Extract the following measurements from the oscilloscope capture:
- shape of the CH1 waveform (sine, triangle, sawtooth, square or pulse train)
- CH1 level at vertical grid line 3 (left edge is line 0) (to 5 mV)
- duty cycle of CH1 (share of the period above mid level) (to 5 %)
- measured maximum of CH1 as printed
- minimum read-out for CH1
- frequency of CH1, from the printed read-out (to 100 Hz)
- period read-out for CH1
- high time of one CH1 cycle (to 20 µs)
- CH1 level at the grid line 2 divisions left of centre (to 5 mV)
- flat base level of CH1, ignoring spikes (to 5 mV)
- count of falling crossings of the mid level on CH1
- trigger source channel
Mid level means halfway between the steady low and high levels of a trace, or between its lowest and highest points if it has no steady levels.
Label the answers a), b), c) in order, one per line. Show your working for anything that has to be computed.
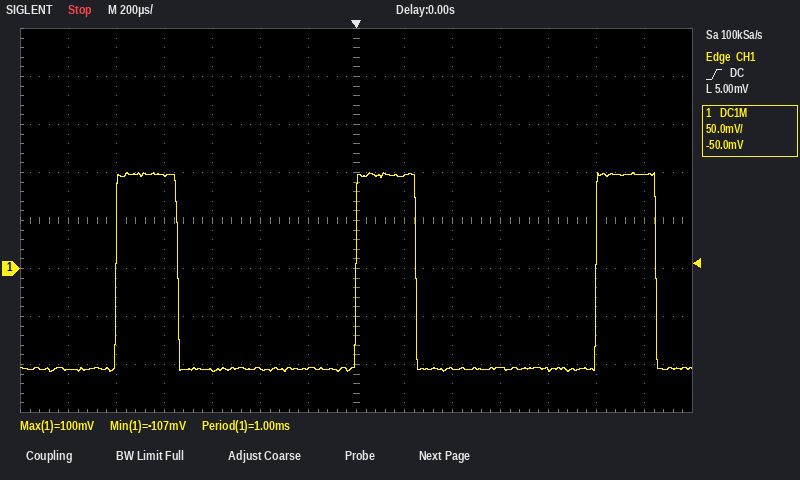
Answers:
a) pulse train
b) 95 mV
c) 25 %
d) 100 mV
e) -107 mV
f) 1 / 1.00 ms ≈ 1.0 kHz
g) 1.00 ms
h) 260 µs
i) -105 mV
j) -105 mV
k) 3
l) CH1
